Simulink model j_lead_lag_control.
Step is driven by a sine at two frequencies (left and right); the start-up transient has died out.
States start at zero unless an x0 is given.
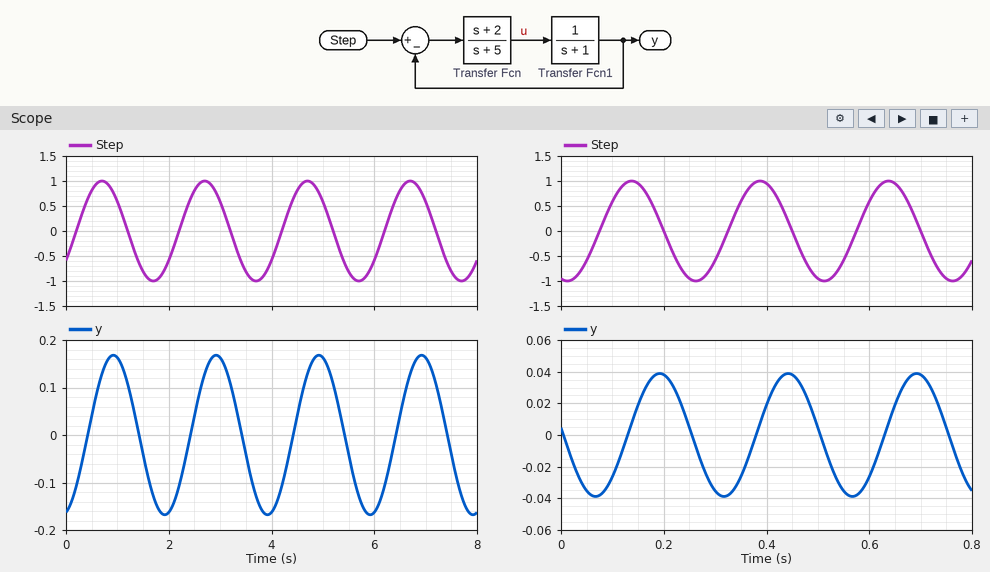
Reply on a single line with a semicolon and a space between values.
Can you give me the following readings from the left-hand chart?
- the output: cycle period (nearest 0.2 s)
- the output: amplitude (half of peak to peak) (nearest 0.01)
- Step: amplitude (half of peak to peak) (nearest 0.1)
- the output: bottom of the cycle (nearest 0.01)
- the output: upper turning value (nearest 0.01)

2.0 s; 0.17; 1.0; -0.17; 0.17
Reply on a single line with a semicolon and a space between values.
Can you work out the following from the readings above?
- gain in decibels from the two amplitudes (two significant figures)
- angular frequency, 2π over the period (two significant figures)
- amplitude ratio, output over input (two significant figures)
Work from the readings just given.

-15 dB; 3.1 rad/s; 0.17
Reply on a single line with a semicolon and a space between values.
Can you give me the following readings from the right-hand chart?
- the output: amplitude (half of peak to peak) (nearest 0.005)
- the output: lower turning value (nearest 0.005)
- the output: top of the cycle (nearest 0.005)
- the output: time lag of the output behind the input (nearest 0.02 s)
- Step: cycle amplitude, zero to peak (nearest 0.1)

0.040; -0.040; 0.040; 0.06 s; 1.0
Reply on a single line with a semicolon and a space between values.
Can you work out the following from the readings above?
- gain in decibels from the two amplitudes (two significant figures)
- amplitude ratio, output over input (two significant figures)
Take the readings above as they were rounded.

-28 dB; 0.040
